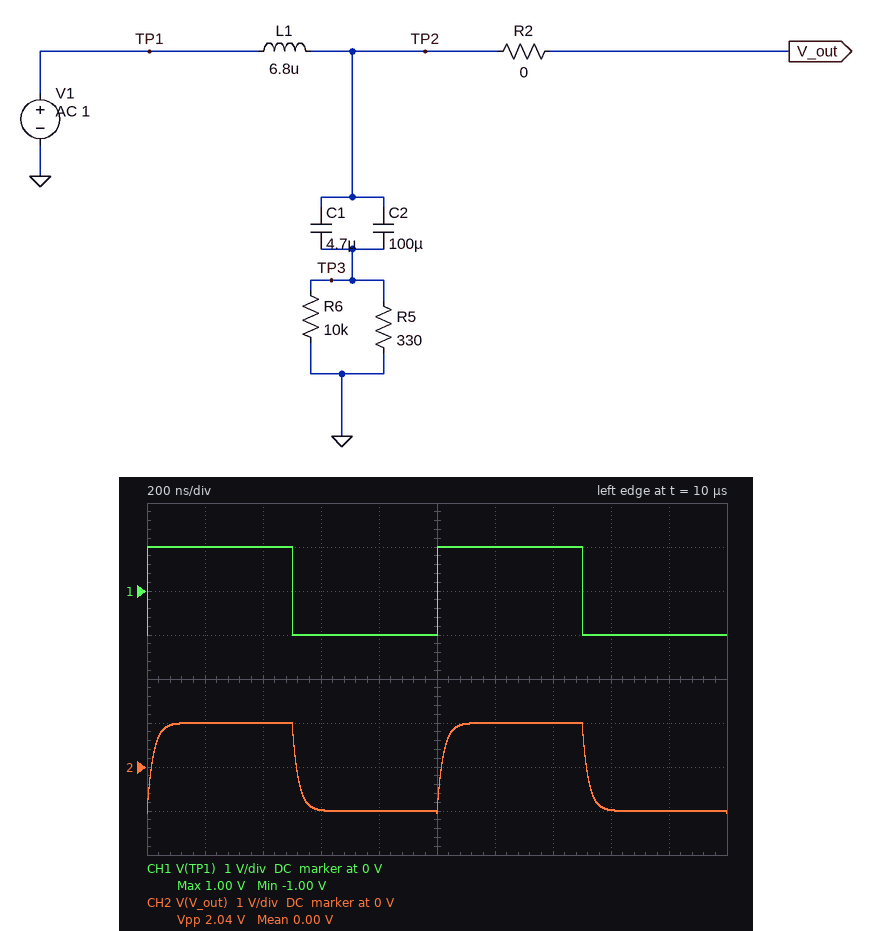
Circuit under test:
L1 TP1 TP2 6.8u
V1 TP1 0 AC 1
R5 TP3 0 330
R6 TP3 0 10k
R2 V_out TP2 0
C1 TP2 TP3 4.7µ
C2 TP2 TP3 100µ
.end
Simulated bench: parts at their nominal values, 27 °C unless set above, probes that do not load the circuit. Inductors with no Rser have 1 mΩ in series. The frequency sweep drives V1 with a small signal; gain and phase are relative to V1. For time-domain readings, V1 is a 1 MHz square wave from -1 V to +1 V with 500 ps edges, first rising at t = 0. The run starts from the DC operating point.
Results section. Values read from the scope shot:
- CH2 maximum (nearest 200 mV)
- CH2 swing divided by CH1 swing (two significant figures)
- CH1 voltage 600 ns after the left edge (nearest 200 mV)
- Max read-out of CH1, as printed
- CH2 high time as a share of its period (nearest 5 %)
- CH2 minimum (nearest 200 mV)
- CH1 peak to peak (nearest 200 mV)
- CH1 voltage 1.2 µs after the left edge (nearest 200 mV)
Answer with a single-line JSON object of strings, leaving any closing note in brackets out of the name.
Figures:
{"CH2 maximum": "1.0 V", "CH2 swing divided by CH1 swing": "1.0", "CH1 voltage 600 ns after the left edge": "-1.0 V", "Max read-out of CH1, as printed": "1.00 V", "CH2 high time as a share of its period": "50 %", "CH2 minimum": "-1.0 V", "CH1 peak to peak": "2.0 V", "CH1 voltage 1.2 µs after the left edge": "1.0 V"}
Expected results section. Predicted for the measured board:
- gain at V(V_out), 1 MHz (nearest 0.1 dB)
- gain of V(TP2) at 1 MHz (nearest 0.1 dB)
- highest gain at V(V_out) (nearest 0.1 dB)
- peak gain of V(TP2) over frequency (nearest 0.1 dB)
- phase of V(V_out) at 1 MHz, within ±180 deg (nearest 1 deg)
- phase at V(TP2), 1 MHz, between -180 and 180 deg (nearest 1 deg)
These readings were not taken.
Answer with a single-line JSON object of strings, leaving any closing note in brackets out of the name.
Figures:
{"gain at V(V_out), 1 MHz": "-0.1 dB", "gain of V(TP2) at 1 MHz": "-0.1 dB", "highest gain at V(V_out)": "0 dB", "peak gain of V(TP2) over frequency": "0 dB", "phase of V(V_out) at 1 MHz, within ±180 deg": "-8 deg", "phase at V(TP2), 1 MHz, between -180 and 180 deg": "-8 deg"}
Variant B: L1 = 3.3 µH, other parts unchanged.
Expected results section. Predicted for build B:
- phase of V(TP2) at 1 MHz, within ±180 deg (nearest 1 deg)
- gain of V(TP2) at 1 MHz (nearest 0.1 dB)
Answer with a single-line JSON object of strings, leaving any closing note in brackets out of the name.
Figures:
{"phase of V(TP2) at 1 MHz, within ±180 deg": "-4 deg", "gain of V(TP2) at 1 MHz": "0 dB"}
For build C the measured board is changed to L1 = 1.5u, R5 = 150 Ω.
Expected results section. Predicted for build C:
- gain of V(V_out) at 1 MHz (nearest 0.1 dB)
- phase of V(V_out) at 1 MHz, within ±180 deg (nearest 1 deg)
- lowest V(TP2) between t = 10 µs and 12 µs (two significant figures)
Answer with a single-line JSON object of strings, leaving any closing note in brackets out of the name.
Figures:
{"gain of V(V_out) at 1 MHz": "0 dB", "phase of V(V_out) at 1 MHz, within ±180 deg": "-4 deg", "lowest V(TP2) between t = 10 µs and 12 µs": "-1.0 V"}
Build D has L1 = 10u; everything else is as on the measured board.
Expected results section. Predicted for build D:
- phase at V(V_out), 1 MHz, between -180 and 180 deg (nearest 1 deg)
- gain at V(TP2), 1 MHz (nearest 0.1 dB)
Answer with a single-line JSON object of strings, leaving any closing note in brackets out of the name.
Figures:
{"phase at V(V_out), 1 MHz, between -180 and 180 deg": "-11 deg", "gain at V(TP2), 1 MHz": "-0.2 dB"}
